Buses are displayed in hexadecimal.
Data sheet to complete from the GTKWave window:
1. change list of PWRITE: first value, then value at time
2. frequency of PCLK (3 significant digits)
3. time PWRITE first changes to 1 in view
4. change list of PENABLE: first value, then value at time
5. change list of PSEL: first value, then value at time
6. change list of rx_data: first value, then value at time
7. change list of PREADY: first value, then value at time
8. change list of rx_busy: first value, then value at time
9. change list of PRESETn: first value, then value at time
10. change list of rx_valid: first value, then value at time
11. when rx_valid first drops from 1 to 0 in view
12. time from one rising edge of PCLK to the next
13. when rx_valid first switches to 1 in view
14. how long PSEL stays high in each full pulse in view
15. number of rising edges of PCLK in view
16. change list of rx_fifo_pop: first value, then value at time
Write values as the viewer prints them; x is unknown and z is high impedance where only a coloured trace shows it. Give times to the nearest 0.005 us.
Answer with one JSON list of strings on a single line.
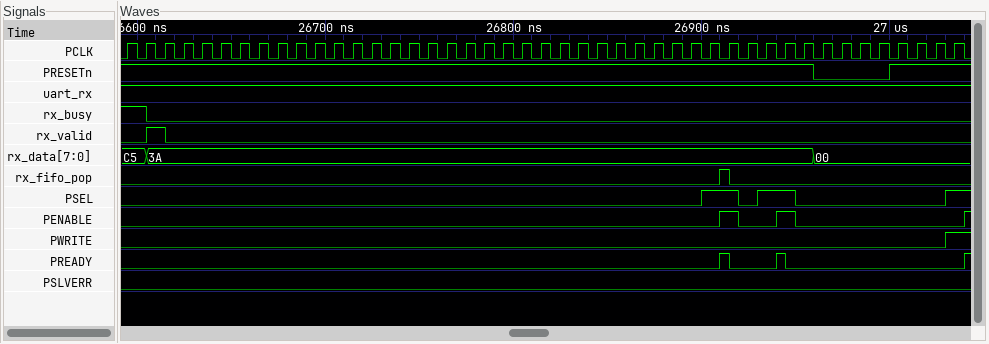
["0, 1 at 27.03 us", "100 MHz", "27.03 us", "0, 1 at 26.91 us, 0 at 26.92 us, 1 at 26.94 us, 0 at 26.95 us, 1 at 27.04 us", "0, 1 at 26.9 us, 0 at 26.92 us, 1 at 26.93 us, 0 at 26.95 us, 1 at 27.03 us", "C5, 3A at 26.605 us, 00 at 26.96 us", "0, 1 at 26.91 us, 0 at 26.915 us, 1 at 26.94 us, 0 at 26.945 us, 1 at 27.04 us", "1, 0 at 26.605 us", "1, 0 at 26.96 us, 1 at 27 us", "0, 1 at 26.605 us, 0 at 26.615 us", "26.615 us", "0.01 us", "26.605 us", "0.02 us, 0.02 us", "45", "0, 1 at 26.91 us, 0 at 26.915 us"]
